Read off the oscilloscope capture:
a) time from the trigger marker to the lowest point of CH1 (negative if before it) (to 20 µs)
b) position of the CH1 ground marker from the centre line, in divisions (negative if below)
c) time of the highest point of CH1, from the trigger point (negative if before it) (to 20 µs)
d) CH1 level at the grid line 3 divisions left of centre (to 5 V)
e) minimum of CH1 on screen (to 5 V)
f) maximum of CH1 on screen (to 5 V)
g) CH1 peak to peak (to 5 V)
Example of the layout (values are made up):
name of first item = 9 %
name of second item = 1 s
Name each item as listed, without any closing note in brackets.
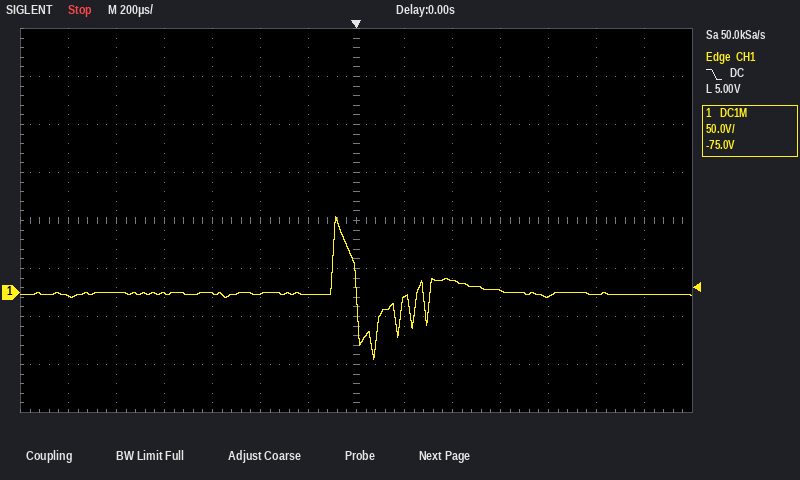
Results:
time from the trigger marker to the lowest point of CH1 (negative if before it) = +80 µs
position of the CH1 ground marker from the centre line, in divisions = -1.5 div
time of the highest point of CH1, from the trigger point (negative if before it) = -80 µs
CH1 level at the grid line 3 divisions left of centre = 0 V
minimum of CH1 on screen = -70 V
maximum of CH1 on screen = 80 V
CH1 peak to peak = 150 V
